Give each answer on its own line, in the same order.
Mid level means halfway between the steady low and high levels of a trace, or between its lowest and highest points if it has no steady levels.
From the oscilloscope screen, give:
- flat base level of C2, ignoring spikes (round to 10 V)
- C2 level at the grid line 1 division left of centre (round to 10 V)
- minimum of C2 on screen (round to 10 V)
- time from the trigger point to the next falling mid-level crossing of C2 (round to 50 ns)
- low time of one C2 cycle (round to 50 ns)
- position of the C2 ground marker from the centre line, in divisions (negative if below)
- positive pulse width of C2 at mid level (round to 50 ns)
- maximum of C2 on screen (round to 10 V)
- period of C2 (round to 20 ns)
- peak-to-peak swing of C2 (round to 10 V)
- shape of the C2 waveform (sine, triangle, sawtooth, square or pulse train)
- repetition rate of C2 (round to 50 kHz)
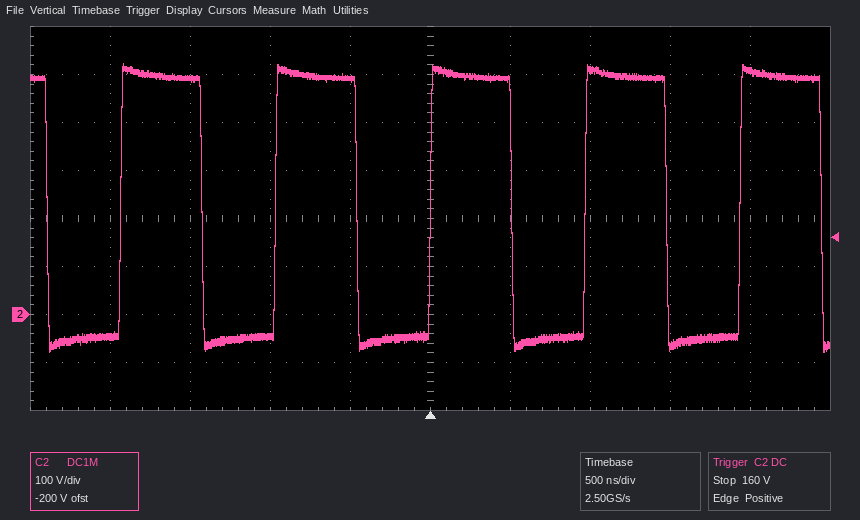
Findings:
-50 V
490 V
-80 V
500 ns
450 ns
-2.0 div
500 ns
520 V
960 ns
600 V
square
1.05 MHz
